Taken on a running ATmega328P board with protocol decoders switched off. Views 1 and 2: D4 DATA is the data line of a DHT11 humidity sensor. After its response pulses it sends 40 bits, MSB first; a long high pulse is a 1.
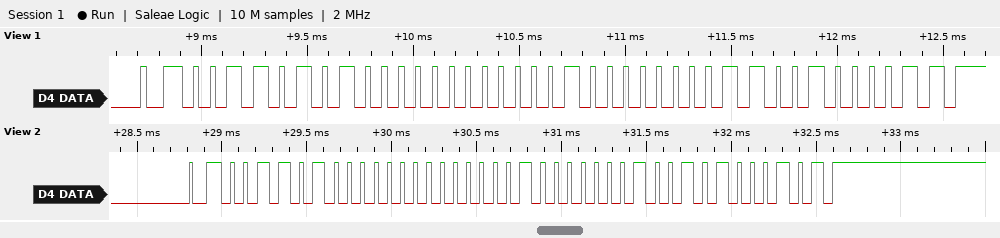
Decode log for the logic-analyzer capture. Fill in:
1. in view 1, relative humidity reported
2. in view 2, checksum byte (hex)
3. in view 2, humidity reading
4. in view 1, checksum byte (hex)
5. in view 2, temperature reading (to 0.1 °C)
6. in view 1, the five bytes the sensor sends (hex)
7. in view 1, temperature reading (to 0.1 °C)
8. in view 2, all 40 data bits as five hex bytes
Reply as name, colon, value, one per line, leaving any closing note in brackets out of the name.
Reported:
in view 1, relative humidity reported: 53 %
in view 2, checksum byte: 0x45
in view 2, humidity reading: 52 %
in view 1, checksum byte: 0x43
in view 2, temperature reading: 8.9 °C
in view 1, the five bytes the sensor sends: 35 00 08 06 43
in view 1, temperature reading: 8.6 °C
in view 2, all 40 data bits as five hex bytes: 34 00 08 09 45
